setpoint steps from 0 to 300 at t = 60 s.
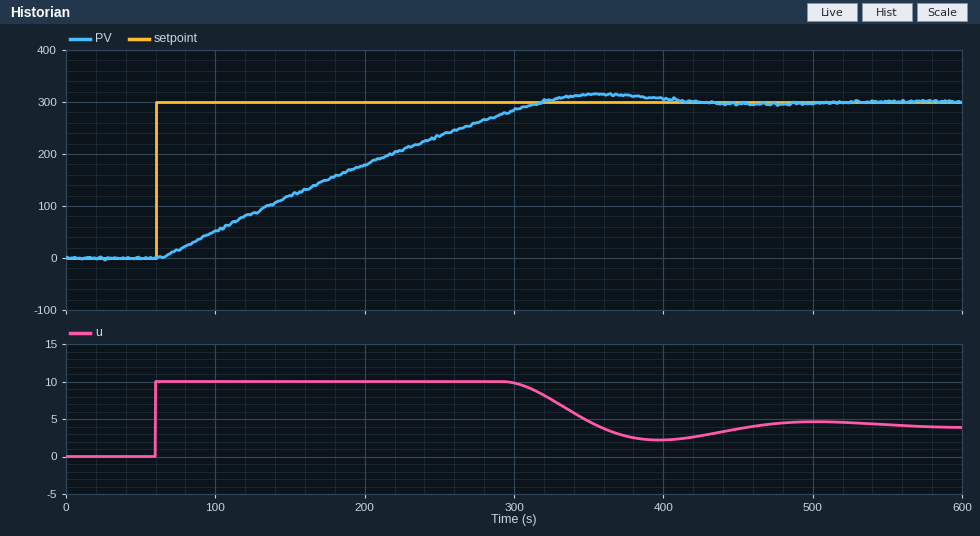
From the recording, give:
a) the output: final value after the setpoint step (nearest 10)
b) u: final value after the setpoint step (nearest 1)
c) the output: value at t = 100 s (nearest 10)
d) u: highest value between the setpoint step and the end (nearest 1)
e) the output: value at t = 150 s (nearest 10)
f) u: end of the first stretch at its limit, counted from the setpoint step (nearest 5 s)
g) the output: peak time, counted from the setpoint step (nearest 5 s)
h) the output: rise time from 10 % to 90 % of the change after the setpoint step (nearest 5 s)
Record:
300
4
50
10
120
240 s
300 s
200 s
